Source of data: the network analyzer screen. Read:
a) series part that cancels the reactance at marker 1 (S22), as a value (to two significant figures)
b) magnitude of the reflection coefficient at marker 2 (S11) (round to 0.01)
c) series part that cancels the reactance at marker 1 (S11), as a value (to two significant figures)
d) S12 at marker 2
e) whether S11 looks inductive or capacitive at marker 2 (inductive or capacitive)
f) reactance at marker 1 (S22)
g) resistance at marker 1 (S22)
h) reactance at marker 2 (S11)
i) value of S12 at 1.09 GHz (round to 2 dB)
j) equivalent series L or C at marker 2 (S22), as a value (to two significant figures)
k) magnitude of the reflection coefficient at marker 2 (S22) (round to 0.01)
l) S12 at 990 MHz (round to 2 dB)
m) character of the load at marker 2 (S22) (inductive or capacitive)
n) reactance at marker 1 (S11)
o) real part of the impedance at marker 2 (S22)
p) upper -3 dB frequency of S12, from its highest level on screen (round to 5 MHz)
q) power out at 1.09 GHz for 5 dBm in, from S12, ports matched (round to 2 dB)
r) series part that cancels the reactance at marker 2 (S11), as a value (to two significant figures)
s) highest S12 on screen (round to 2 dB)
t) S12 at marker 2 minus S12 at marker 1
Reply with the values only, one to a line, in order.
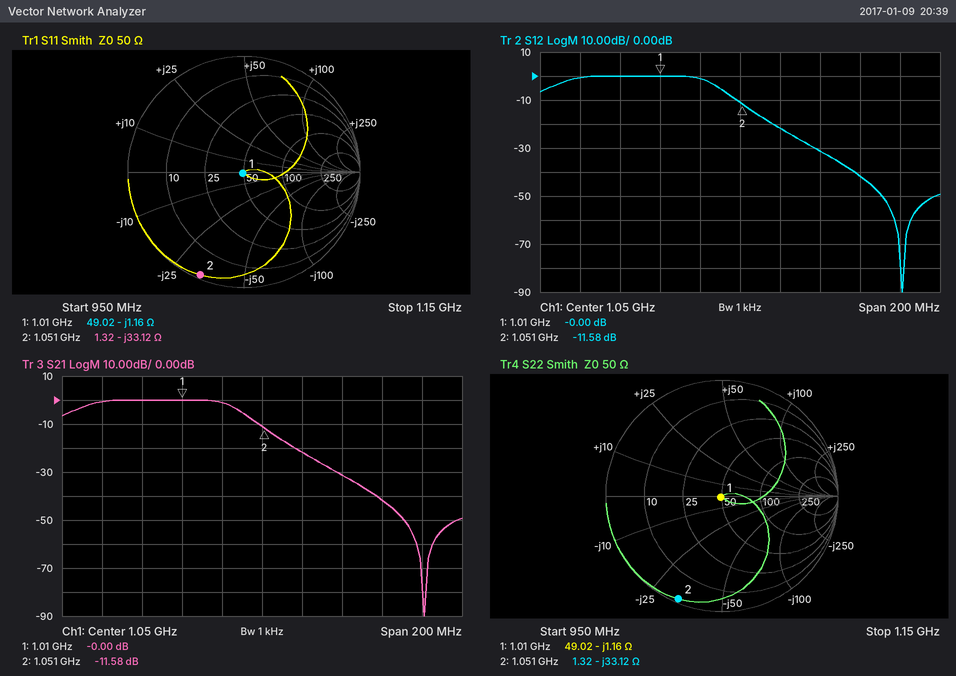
180 pH
0.96
180 pH
-11.58 dB
capacitive
-1.16 Ω
49.02 Ω
-33.12 Ω
-32 dB
4.6 pF
0.96
0 dB
capacitive
-1.16 Ω
1.32 Ω
1.035 GHz
-26 dBm
5.0 nH
0 dB
-11.58 dB
